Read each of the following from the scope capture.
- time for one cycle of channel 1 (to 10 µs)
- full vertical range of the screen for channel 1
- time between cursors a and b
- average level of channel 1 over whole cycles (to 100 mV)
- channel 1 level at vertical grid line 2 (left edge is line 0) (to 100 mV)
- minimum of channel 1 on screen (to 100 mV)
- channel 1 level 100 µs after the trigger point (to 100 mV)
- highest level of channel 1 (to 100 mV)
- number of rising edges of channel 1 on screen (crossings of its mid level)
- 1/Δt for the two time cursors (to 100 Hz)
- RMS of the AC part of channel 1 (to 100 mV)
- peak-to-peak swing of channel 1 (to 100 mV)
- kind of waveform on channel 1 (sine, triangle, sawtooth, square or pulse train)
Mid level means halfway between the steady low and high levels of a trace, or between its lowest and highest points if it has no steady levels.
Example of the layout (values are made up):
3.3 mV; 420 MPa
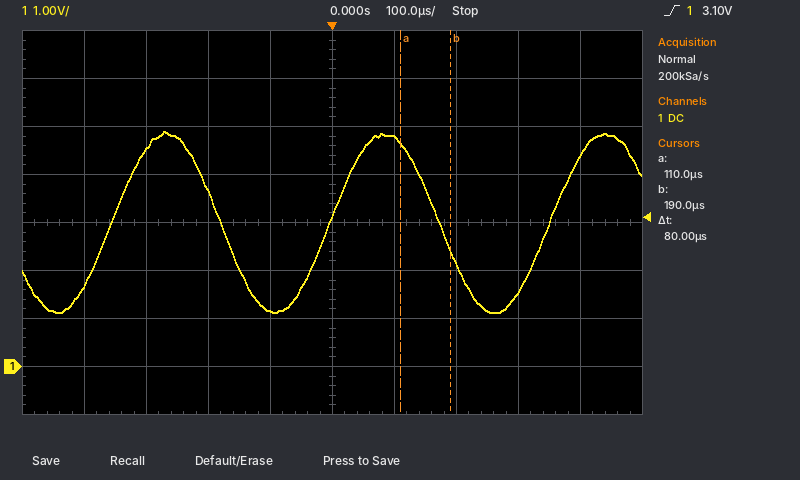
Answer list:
350 µs; 8 V; 80 µs; 3.0 V; 4.5 V; 1.1 V; 4.8 V; 4.9 V; 3; 12.5 kHz; 1.3 V; 3.8 V; sine
